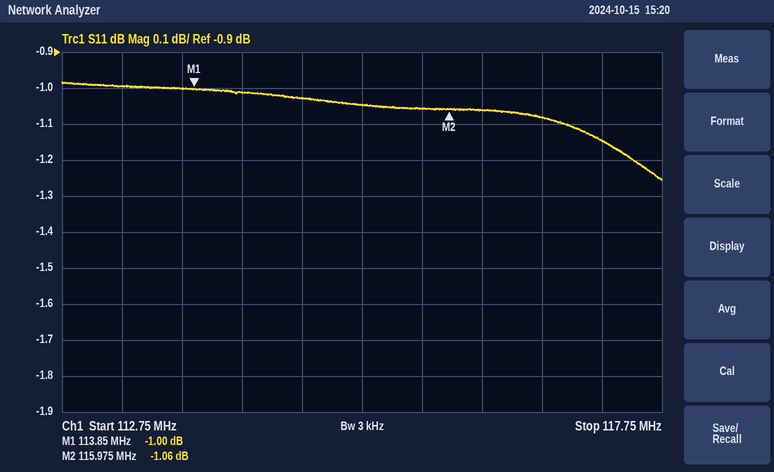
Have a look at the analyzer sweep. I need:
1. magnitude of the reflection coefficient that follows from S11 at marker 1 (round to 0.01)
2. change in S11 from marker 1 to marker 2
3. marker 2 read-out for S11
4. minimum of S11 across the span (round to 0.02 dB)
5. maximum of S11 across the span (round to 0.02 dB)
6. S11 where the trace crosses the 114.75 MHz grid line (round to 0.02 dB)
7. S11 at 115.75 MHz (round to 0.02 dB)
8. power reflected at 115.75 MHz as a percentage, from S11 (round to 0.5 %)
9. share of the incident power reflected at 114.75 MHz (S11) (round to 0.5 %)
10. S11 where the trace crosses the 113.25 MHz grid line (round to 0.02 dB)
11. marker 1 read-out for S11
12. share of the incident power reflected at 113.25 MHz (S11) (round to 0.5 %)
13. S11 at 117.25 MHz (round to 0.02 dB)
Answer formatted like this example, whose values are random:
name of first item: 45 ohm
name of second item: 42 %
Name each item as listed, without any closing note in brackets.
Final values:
magnitude of the reflection coefficient that follows from S11 at marker 1: 0.89
change in S11 from marker 1 to marker 2: -0.06 dB
marker 2 read-out for S11: -1.06 dB
minimum of S11 across the span: -1.26 dB
maximum of S11 across the span: -0.98 dB
S11 where the trace crosses the 114.75 MHz grid line: -1.02 dB
S11 at 115.75 MHz: -1.06 dB
power reflected at 115.75 MHz as a percentage, from S11: 78.5 %
share of the incident power reflected at 114.75 MHz (S11): 79.0 %
S11 where the trace crosses the 113.25 MHz grid line: -1.00 dB
marker 1 read-out for S11: -1.00 dB
share of the incident power reflected at 113.25 MHz (S11): 79.5 %
S11 at 117.25 MHz: -1.14 dB
